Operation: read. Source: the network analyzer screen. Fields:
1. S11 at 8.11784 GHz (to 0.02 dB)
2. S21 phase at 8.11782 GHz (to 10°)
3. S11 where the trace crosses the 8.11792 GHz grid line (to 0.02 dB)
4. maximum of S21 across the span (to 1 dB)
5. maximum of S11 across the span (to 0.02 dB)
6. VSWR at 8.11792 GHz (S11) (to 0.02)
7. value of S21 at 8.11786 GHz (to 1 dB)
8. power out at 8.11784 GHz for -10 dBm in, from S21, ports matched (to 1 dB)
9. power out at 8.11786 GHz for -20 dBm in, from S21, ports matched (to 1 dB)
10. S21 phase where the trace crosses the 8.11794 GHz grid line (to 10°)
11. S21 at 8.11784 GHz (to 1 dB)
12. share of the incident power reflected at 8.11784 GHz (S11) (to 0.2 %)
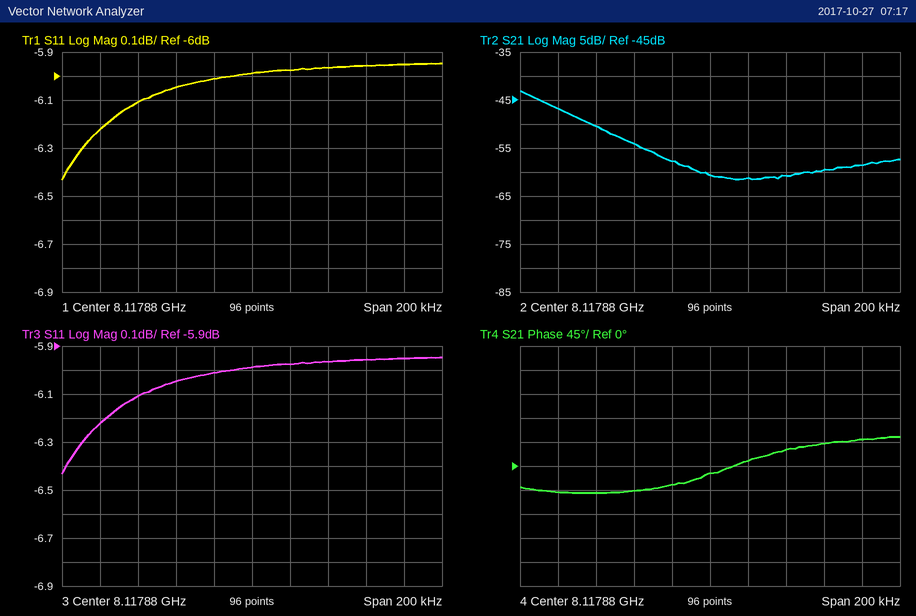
-6.04 dB
-50°
-5.96 dB
-43 dB
-5.94 dB
3.02
-58 dB
-64 dBm
-78 dBm
40°
-54 dB
24.8 %
